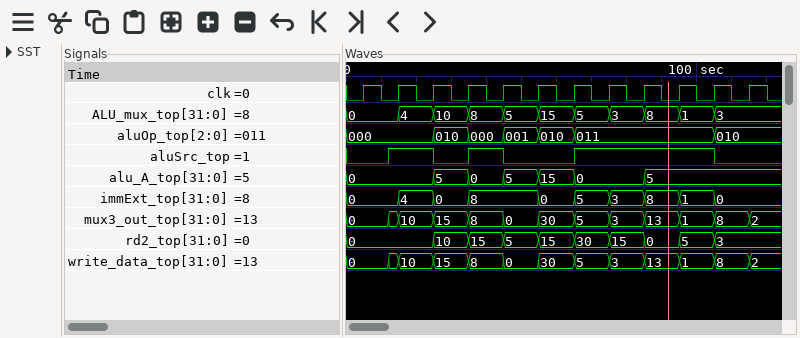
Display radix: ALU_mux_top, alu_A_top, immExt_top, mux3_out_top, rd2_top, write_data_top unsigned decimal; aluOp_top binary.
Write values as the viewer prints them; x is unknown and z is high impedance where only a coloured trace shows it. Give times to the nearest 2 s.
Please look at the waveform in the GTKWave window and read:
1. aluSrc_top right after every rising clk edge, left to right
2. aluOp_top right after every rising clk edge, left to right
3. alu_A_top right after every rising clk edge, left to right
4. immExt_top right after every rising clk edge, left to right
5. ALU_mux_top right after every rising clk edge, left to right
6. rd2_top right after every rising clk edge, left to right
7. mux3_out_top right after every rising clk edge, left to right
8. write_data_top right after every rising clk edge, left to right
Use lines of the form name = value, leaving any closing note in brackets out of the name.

aluSrc_top right after every rising clk edge, left to right = 0 1 0 1 0 0 1 1 1 1 0 0
aluOp_top right after every rising clk edge, left to right = 000, 000, 010, 000, 001, 010, 011, 011, 011, 011, 010, 010
alu_A_top right after every rising clk edge, left to right = 0, 0, 5, 0, 5, 15, 0, 0, 5, 5, 5, 5
immExt_top right after every rising clk edge, left to right = 0, 4, 0, 8, 8, 0, 5, 3, 8, 1, 0, 0
ALU_mux_top right after every rising clk edge, left to right = 0, 4, 10, 8, 5, 15, 5, 3, 8, 1, 3, 3
rd2_top right after every rising clk edge, left to right = 0, 0, 10, 15, 5, 15, 30, 15, 0, 5, 3, 3
mux3_out_top right after every rising clk edge, left to right = 0, 10, 15, 8, 0, 30, 5, 3, 13, 1, 8, 2
write_data_top right after every rising clk edge, left to right = 0, 10, 15, 8, 0, 30, 5, 3, 13, 1, 8, 2
